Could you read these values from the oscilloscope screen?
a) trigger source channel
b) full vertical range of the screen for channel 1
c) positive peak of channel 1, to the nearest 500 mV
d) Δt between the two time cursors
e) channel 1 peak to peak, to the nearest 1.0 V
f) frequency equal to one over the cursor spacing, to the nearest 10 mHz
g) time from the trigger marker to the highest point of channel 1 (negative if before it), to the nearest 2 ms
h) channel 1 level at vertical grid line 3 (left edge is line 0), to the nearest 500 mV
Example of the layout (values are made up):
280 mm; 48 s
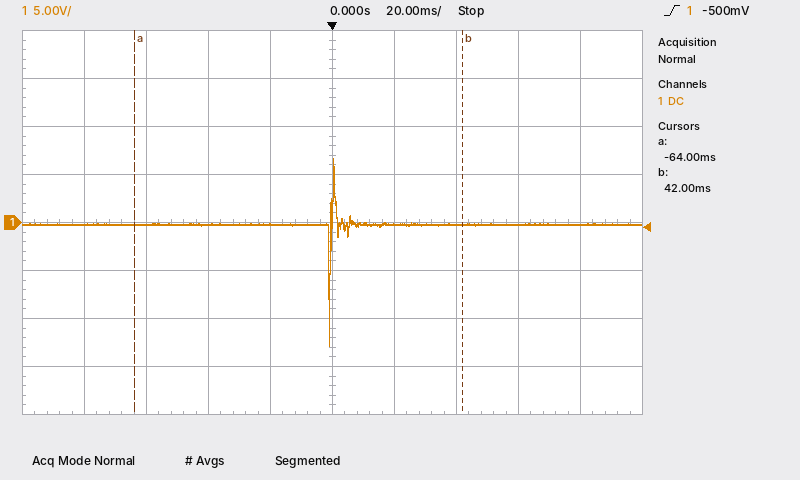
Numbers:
channel 1; 40 V; 6.5 V; 106 ms; 19.0 V; 9.43 Hz; 0 ms; 0.0 V
